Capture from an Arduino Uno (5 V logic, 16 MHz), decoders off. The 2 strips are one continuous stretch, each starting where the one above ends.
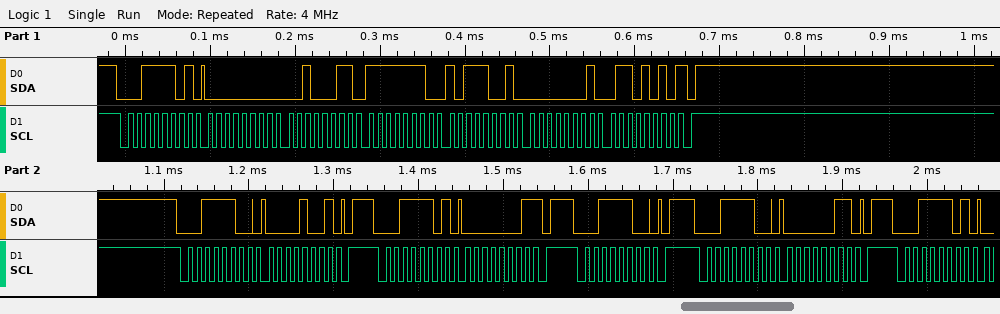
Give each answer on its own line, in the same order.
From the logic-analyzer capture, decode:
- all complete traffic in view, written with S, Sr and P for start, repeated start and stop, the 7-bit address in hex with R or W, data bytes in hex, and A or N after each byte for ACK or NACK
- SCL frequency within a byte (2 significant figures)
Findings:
S 1ER A 00 A 23 A FE A B9 A 01 A 6A N P S 1EW A 09 A P S 1ER A 01 N P S 1EW A P S 1EW A 03 A P S 1ER A
100 kHz
